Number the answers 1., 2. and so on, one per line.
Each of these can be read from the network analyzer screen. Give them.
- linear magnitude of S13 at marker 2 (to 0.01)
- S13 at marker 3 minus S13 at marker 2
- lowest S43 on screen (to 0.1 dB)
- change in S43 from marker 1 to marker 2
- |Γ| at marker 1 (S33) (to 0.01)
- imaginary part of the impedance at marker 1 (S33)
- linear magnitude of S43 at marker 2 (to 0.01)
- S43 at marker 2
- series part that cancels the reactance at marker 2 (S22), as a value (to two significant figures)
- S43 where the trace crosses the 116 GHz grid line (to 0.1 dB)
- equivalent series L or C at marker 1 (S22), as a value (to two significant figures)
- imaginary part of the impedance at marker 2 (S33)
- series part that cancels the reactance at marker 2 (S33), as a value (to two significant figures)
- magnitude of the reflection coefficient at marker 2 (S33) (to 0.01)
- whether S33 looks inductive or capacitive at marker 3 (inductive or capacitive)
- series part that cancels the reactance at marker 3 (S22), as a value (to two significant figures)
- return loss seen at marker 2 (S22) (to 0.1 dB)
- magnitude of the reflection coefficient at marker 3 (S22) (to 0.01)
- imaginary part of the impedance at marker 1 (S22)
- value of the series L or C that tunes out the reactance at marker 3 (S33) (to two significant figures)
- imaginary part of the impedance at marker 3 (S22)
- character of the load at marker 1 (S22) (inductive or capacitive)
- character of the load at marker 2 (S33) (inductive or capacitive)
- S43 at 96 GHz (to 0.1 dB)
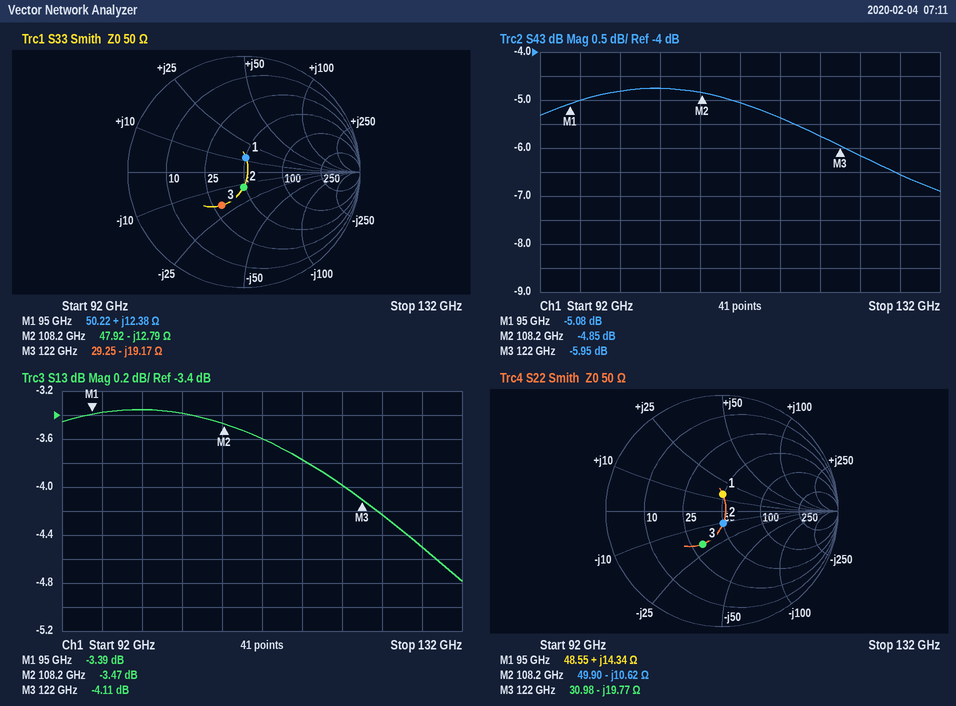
1. 0.67
2. -0.64 dB
3. -6.9 dB
4. 0.23 dB
5. 0.12
6. +12.38 Ω
7. 0.57
8. -4.85 dB
9. 16 pH
10. -5.4 dB
11. 24 pH
12. -12.79 Ω
13. 19 pH
14. 0.13
15. capacitive
16. 26 pH
17. 19.5 dB
18. 0.33
19. +14.34 Ω
20. 25 pH
21. -19.77 Ω
22. inductive
23. capacitive
24. -5.0 dB
